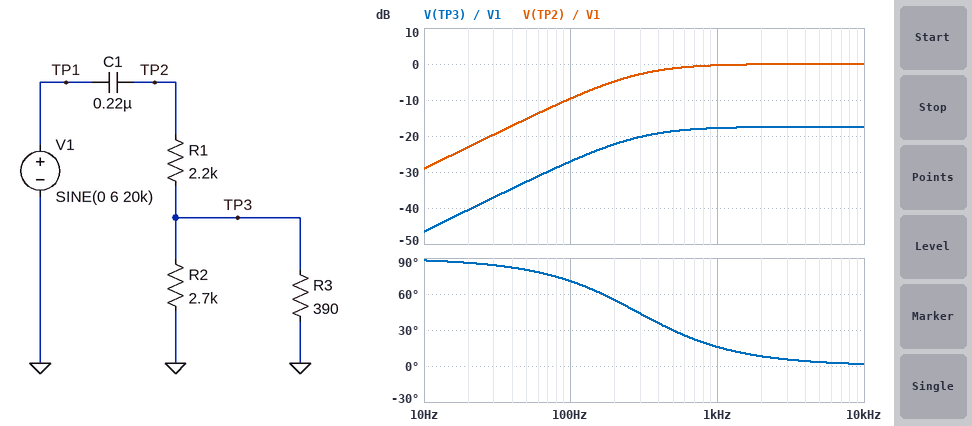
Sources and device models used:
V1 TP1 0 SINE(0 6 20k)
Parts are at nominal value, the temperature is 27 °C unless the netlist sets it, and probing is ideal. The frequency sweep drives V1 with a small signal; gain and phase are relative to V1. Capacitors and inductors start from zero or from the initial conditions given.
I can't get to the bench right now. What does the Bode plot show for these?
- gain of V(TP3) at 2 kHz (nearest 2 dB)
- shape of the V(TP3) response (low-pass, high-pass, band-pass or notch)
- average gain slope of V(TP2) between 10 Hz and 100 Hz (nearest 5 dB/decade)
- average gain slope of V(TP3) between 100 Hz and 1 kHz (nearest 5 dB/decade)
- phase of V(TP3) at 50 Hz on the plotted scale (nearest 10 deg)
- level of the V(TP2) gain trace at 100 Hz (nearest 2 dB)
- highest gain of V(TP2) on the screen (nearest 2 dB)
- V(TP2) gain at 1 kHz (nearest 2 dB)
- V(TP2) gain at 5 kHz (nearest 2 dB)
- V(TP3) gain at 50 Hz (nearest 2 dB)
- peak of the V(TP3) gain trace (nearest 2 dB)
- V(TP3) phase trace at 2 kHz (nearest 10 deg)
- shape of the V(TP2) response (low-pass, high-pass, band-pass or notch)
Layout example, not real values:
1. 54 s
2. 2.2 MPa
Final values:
1. -18 dB
2. high-pass
3. 20 dB/decade
4. 10 dB/decade
5. 80 deg
6. -10 dB
7. 0 dB
8. 0 dB
9. 0 dB
10. -32 dB
11. -18 dB
12. 10 deg
13. high-pass
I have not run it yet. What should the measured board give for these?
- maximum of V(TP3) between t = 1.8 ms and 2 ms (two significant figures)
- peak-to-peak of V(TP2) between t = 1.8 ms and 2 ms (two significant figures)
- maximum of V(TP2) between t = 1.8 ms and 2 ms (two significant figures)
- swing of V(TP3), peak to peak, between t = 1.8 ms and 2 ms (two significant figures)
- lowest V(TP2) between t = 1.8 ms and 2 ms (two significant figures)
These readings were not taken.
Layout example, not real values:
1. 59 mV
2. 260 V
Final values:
1. 800 mV
2. 12 V
3. 6.0 V
4. 1.6 V
5. -6.0 V
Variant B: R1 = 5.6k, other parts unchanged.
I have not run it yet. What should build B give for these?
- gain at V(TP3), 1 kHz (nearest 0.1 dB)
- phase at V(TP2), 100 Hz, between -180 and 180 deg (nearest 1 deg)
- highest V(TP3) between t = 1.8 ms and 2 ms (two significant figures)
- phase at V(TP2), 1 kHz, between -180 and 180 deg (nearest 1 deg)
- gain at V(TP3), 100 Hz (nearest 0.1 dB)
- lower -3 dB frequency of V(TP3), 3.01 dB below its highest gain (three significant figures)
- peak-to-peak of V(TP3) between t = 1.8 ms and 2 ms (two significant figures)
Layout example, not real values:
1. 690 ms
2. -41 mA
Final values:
1. -24.9 dB
2. 51 deg
3. 340 mV
4. 7 deg
5. -28.8 dB
6. 122 Hz
7. 690 mV
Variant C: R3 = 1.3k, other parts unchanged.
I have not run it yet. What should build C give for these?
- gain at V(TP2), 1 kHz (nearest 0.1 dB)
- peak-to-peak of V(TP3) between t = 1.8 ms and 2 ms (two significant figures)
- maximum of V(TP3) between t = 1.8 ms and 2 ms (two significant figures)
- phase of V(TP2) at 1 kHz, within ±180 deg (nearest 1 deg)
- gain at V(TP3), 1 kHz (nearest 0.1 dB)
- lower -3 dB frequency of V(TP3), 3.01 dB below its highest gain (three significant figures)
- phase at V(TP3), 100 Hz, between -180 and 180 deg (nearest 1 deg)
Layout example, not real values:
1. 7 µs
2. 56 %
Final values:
1. -0.2 dB
2. 3.4 V
3. 1.7 V
4. 13 deg
5. -11.1 dB
6. 235 Hz
7. 67 deg
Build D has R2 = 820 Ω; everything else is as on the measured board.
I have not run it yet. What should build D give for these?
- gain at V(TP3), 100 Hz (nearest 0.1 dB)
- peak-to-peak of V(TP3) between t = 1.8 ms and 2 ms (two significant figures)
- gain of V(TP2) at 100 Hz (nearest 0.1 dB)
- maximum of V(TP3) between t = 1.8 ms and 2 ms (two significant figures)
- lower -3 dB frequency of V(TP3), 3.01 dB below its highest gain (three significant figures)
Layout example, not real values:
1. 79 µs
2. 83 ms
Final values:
1. -29.2 dB
2. 1.3 V
3. -9.8 dB
4. 640 mV
5. 294 Hz
